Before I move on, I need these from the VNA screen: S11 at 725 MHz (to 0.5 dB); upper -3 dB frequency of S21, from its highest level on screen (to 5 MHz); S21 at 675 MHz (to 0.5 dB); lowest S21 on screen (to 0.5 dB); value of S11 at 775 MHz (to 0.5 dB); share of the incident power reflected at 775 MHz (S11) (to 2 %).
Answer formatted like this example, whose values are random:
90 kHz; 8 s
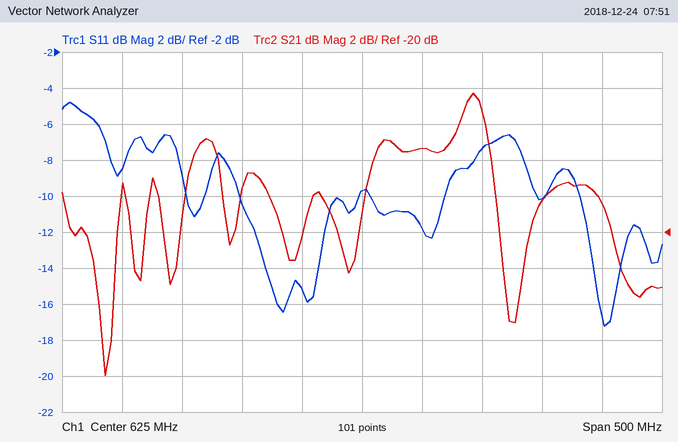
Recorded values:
-7.5 dB; 730 MHz; -15.5 dB; -28.0 dB; -10.0 dB; 10 %
